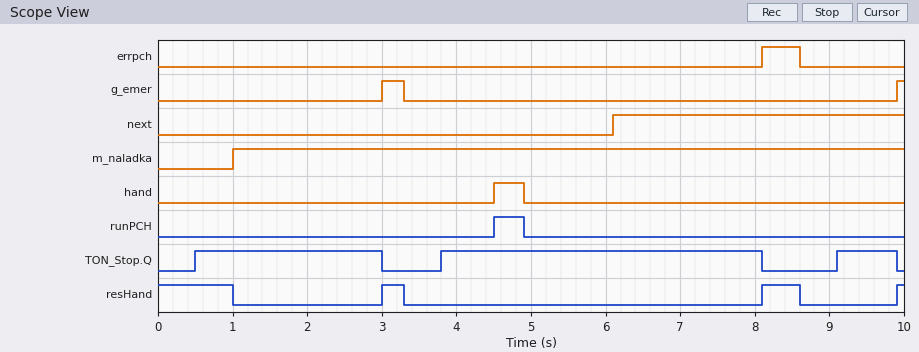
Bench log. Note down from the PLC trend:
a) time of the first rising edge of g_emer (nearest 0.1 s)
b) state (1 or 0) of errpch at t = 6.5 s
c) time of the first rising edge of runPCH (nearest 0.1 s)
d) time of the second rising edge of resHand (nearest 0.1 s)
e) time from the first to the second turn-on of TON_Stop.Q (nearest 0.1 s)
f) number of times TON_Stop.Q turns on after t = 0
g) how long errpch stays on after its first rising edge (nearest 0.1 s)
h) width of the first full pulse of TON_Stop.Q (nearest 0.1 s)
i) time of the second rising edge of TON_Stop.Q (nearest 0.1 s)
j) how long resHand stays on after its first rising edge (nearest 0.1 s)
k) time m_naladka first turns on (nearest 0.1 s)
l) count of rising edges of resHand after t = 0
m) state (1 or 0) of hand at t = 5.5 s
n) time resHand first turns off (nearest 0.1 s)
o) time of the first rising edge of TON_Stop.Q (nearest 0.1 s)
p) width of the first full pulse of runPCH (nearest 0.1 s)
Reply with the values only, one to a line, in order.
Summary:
3.0 s
0
4.5 s
8.1 s
3.3 s
3
0.5 s
2.5 s
3.8 s
0.3 s
1.0 s
3
0
1.0 s
0.5 s
0.4 s
